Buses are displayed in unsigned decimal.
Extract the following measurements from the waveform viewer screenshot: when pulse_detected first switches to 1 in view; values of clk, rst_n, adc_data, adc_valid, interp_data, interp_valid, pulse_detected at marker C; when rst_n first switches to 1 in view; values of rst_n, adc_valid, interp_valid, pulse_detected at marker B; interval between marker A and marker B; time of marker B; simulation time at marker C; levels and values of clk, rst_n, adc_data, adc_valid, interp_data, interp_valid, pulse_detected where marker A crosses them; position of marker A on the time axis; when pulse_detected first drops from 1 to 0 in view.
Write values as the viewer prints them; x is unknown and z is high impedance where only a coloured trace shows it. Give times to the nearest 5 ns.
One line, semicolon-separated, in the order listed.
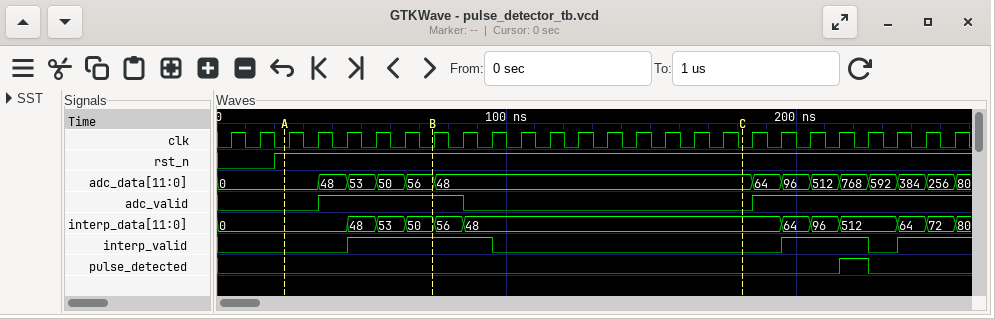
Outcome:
215 ns; clk=0, rst_n=1, adc_data=48, adc_valid=0, interp_data=48, interp_valid=0, pulse_detected=0; 20 ns; rst_n=1, adc_valid=1, interp_valid=1, pulse_detected=0; 50 ns; 75 ns; 180 ns; clk=0, rst_n=1, adc_data=0, adc_valid=0, interp_data=0, interp_valid=0, pulse_detected=0; 25 ns; 225 ns
